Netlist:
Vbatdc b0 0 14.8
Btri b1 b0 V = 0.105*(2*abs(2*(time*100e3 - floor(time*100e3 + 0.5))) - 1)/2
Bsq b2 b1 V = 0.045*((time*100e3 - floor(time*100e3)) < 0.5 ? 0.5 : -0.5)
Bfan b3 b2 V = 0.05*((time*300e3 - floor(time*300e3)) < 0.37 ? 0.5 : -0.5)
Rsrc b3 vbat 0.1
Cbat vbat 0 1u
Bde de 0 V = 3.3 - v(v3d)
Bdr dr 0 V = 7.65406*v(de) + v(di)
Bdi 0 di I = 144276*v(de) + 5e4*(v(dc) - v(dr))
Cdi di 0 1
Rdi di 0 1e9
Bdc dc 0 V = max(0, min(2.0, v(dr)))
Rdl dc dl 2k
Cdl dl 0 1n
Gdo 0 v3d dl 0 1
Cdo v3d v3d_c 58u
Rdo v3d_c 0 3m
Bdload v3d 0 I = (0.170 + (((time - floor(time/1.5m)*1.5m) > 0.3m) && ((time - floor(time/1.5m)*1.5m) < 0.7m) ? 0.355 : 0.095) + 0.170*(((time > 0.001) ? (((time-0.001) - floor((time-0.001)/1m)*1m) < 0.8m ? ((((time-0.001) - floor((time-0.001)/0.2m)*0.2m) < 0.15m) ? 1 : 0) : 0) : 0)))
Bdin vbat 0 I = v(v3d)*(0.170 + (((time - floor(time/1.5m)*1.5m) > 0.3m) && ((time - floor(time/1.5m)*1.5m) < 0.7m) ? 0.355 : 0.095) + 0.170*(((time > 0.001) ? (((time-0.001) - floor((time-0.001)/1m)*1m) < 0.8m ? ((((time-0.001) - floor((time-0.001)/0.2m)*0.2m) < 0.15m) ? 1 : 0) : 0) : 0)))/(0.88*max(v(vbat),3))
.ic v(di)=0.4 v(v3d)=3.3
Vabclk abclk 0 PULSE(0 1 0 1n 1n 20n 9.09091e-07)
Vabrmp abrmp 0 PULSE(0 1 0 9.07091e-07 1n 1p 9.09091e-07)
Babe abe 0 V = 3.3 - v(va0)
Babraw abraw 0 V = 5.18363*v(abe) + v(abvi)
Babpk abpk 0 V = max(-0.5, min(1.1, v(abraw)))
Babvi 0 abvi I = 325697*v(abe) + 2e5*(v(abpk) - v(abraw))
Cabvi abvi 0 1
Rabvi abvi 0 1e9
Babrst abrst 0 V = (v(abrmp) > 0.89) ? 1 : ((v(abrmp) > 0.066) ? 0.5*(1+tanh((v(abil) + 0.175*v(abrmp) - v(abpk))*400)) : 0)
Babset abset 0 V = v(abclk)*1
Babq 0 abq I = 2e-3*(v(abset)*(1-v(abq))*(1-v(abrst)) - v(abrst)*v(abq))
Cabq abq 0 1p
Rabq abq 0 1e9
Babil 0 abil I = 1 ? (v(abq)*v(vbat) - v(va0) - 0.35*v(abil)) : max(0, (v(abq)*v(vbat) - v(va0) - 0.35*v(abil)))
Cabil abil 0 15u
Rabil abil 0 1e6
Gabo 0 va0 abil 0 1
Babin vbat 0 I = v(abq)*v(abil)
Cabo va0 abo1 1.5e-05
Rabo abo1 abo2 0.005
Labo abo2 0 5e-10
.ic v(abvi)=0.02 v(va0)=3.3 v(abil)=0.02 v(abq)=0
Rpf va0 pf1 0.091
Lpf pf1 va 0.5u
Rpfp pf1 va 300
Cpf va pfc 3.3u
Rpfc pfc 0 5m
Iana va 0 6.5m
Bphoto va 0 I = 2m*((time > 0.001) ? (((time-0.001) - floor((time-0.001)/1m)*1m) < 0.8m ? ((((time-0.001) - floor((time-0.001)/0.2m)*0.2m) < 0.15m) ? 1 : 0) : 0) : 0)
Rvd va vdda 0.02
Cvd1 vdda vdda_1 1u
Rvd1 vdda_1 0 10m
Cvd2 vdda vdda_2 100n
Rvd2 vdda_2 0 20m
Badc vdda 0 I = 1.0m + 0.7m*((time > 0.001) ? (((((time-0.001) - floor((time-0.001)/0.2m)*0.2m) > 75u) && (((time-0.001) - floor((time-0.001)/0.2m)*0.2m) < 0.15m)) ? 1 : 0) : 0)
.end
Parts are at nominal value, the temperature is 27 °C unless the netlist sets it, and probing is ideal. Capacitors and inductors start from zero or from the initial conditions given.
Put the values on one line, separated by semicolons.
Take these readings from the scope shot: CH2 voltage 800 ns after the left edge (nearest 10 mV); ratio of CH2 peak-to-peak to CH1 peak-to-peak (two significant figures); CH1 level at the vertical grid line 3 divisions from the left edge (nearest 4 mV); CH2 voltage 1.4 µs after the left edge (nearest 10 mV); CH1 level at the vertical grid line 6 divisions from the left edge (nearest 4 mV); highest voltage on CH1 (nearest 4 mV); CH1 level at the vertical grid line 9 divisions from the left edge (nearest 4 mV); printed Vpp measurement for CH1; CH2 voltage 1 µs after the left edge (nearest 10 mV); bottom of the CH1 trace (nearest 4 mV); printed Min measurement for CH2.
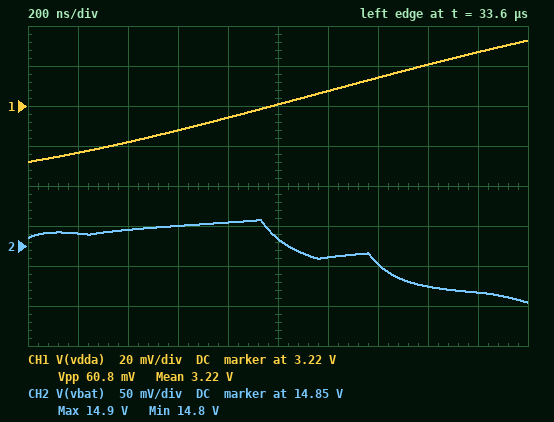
14.88 V; 1.7; 3.208 V; 14.83 V; 3.228 V; 3.252 V; 3.248 V; 60.8 mV; 14.86 V; 3.192 V; 14.8 V
